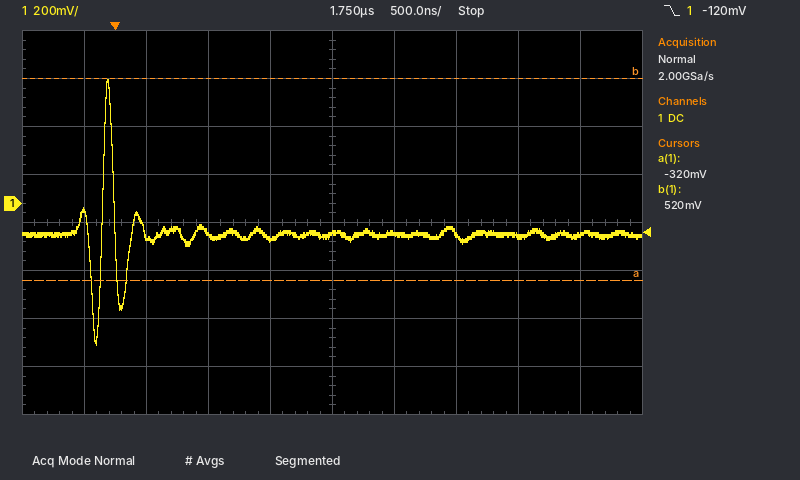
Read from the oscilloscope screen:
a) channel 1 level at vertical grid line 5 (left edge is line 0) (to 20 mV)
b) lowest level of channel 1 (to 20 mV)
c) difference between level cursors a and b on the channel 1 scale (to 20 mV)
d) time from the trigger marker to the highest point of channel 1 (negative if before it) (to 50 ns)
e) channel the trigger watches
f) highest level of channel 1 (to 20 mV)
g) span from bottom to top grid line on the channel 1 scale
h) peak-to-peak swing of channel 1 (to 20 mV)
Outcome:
-120 mV
-580 mV
840 mV
-50 ns
channel 1
520 mV
1.6 V
1.10 V
